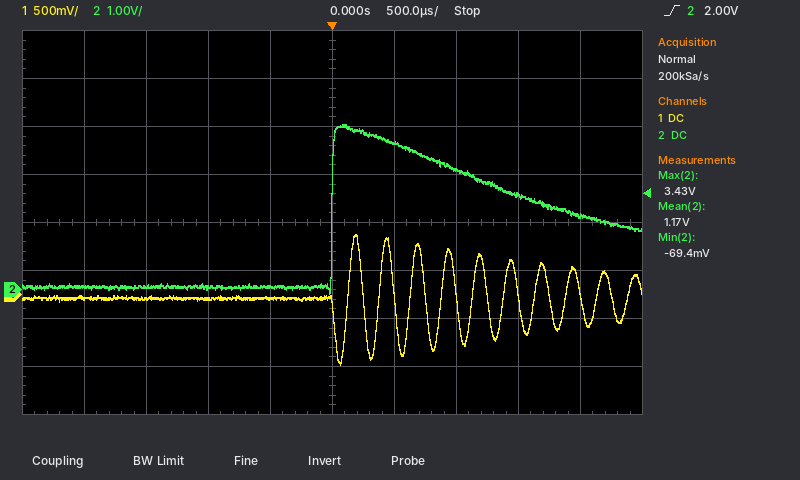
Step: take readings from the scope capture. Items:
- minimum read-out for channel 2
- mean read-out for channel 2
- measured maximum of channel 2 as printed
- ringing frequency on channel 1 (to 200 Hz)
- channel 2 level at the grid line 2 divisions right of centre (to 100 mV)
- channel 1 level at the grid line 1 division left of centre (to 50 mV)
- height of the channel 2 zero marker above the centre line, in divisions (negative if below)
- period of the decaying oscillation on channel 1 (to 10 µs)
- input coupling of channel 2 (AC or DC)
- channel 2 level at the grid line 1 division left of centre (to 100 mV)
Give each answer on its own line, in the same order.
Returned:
-69.4 mV
1.17 V
3.43 V
4.0 kHz
2.5 V
-50 mV
-1.4 div
250 µs
DC
100 mV
